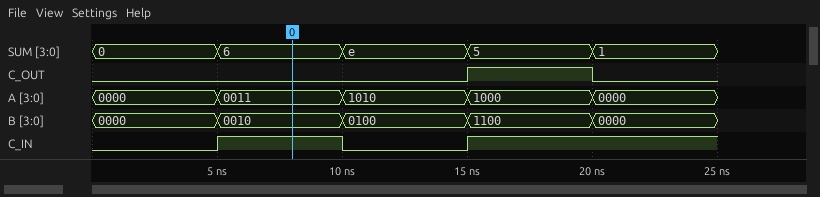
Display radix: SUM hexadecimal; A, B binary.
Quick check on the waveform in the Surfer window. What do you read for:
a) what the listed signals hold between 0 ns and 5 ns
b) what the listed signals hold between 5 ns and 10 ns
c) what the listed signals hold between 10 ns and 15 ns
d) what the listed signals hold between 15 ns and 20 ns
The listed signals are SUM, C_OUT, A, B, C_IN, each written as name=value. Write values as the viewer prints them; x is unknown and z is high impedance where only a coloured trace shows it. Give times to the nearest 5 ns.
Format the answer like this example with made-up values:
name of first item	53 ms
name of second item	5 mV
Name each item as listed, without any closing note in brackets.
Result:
what the listed signals hold between 0 ns and 5 ns	SUM=0, C_OUT=0, A=0000, B=0000, C_IN=0
what the listed signals hold between 5 ns and 10 ns	SUM=6, C_OUT=0, A=0011, B=0010, C_IN=1
what the listed signals hold between 10 ns and 15 ns	SUM=e, C_OUT=0, A=1010, B=0100, C_IN=0
what the listed signals hold between 15 ns and 20 ns	SUM=5, C_OUT=1, A=1000, B=1100, C_IN=1
